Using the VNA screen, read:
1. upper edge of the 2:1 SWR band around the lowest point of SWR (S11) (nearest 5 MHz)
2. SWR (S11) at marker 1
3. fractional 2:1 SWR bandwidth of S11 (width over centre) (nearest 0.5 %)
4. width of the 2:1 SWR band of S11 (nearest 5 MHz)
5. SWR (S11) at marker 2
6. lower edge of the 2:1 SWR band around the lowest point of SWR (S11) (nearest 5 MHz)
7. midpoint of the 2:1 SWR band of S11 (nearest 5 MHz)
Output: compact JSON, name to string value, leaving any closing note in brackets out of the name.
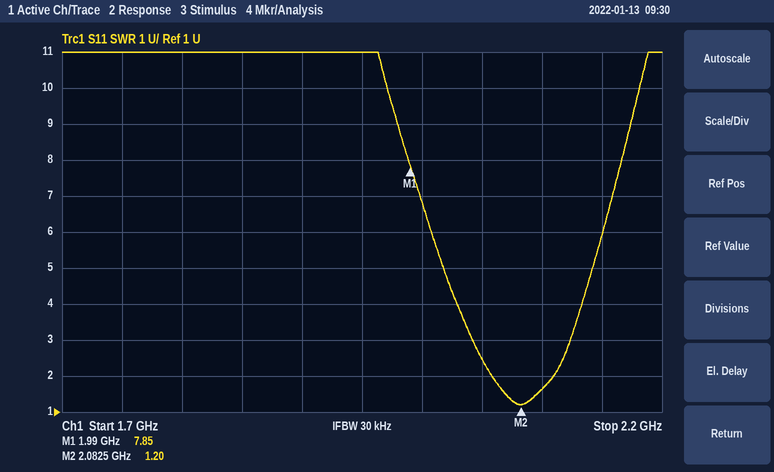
{"upper edge of the 2:1 SWR band around the lowest point of SWR (S11)": "2.110 GHz", "SWR (S11) at marker 1": "7.85", "fractional 2:1 SWR bandwidth of S11 (width over centre)": "2.5 %", "width of the 2:1 SWR band of S11": "50 MHz", "SWR (S11) at marker 2": "1.20", "lower edge of the 2:1 SWR band around the lowest point of SWR (S11)": "2.060 GHz", "midpoint of the 2:1 SWR band of S11": "2.085 GHz"}
